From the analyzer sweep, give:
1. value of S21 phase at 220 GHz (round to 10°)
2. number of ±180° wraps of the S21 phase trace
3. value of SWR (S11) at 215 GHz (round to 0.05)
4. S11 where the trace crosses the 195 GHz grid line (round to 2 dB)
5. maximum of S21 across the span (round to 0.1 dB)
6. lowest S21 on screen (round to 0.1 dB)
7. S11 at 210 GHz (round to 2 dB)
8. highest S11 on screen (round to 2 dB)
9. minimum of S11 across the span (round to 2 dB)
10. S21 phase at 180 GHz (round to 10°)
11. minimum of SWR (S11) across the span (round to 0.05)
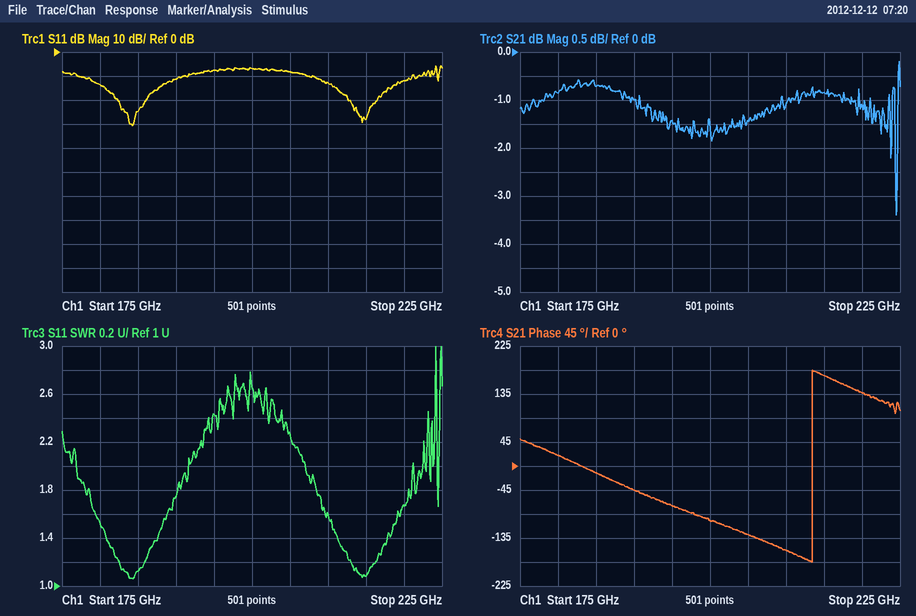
140°
1
1.10
-8 dB
-0.2 dB
-3.4 dB
-12 dB
-6 dB
-30 dB
20°
1.05
